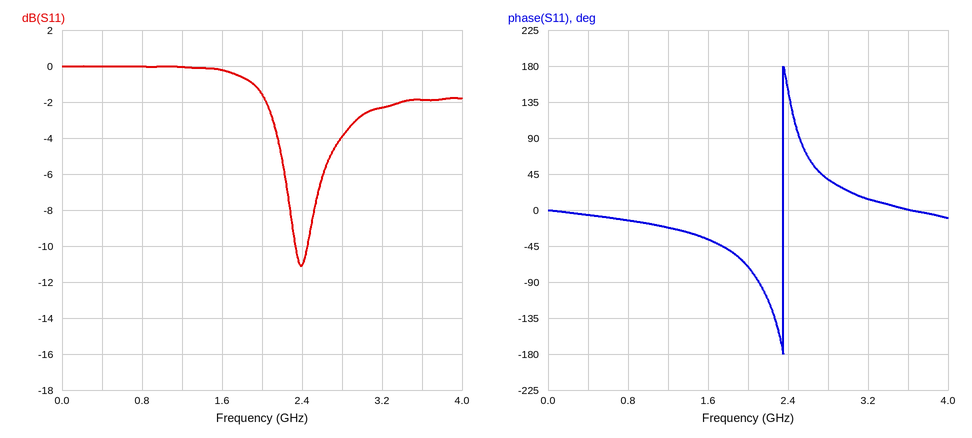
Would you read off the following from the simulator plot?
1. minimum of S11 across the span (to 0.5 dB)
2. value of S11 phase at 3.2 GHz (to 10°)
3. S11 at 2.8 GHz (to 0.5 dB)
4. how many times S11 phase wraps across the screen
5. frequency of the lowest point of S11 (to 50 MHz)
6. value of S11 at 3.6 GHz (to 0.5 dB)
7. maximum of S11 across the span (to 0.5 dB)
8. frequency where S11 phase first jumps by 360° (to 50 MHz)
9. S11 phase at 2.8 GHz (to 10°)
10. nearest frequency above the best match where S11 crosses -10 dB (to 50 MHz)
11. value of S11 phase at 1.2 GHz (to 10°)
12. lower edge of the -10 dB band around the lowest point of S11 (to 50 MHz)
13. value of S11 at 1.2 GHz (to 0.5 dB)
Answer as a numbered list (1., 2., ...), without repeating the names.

1. -11.0 dB
2. 10°
3. -4.0 dB
4. 1
5. 2.40 GHz
6. -2.0 dB
7. 0.0 dB
8. 2.35 GHz
9. 40°
10. 2.45 GHz
11. -20°
12. 2.35 GHz
13. 0.0 dB
